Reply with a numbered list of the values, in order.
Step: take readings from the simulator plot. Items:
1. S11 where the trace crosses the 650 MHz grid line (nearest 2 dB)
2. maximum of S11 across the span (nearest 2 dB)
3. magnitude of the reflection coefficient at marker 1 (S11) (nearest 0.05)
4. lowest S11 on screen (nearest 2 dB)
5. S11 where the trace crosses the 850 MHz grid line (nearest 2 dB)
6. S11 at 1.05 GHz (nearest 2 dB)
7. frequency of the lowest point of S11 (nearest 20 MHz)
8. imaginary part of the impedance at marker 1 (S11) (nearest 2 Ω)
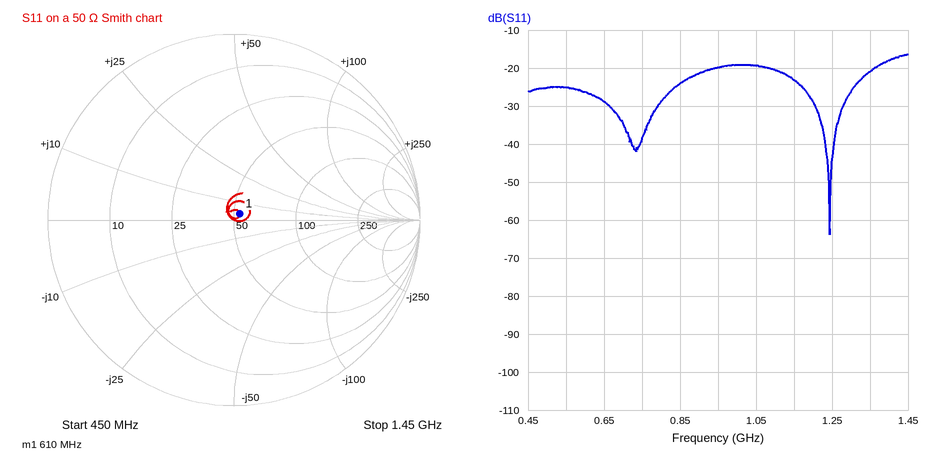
1. -28 dB
2. -16 dB
3. 0.05
4. -64 dB
5. -24 dB
6. -20 dB
7. 1.24 GHz
8. +4 Ω
